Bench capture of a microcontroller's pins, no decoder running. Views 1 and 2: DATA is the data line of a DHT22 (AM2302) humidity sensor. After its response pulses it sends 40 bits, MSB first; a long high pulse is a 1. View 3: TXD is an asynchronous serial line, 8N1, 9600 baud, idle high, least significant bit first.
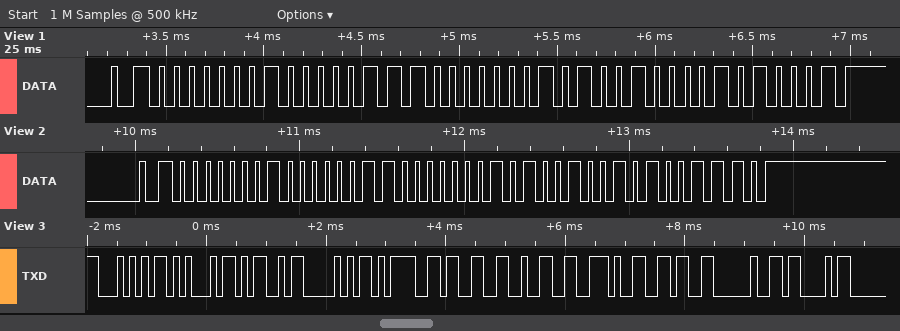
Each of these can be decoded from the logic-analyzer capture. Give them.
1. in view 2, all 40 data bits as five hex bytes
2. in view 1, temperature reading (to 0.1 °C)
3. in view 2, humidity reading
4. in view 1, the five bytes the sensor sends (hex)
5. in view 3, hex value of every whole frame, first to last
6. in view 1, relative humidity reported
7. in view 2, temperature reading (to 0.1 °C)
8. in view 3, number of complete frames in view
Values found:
01 03 01 49 4E
32.8 °C
25.9 %
01 07 01 48 51
54 45 4D 50 3D 33 32 2E 36 20 43
26.3 %
32.9 °C
11
